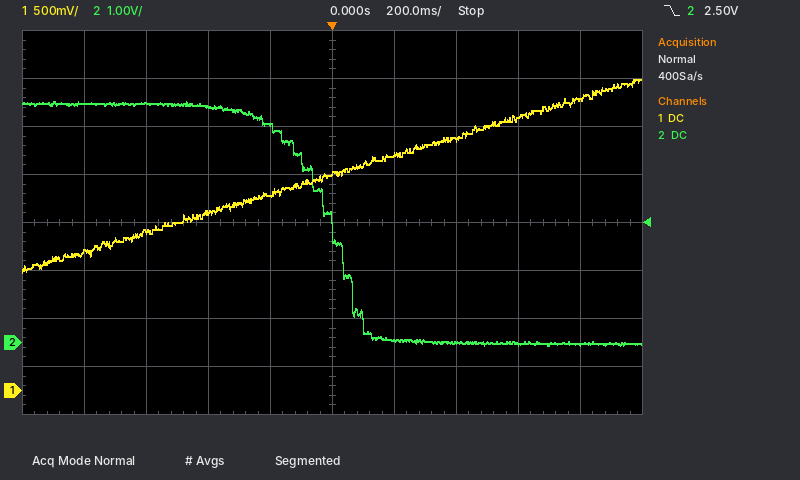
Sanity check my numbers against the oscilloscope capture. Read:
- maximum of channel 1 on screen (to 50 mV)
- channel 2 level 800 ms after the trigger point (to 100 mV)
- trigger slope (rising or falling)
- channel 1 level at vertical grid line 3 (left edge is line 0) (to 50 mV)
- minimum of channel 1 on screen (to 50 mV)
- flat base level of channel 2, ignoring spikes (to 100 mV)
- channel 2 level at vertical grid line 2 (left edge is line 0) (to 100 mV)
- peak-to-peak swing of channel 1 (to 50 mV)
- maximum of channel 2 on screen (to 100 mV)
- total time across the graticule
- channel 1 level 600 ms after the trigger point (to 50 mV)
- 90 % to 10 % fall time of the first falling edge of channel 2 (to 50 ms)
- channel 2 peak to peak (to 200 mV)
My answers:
3.25 V
0.0 V
falling
1.85 V
1.25 V
0.0 V
5.0 V
2.00 V
5.0 V
2 s
2.85 V
300 ms
5.0 V
